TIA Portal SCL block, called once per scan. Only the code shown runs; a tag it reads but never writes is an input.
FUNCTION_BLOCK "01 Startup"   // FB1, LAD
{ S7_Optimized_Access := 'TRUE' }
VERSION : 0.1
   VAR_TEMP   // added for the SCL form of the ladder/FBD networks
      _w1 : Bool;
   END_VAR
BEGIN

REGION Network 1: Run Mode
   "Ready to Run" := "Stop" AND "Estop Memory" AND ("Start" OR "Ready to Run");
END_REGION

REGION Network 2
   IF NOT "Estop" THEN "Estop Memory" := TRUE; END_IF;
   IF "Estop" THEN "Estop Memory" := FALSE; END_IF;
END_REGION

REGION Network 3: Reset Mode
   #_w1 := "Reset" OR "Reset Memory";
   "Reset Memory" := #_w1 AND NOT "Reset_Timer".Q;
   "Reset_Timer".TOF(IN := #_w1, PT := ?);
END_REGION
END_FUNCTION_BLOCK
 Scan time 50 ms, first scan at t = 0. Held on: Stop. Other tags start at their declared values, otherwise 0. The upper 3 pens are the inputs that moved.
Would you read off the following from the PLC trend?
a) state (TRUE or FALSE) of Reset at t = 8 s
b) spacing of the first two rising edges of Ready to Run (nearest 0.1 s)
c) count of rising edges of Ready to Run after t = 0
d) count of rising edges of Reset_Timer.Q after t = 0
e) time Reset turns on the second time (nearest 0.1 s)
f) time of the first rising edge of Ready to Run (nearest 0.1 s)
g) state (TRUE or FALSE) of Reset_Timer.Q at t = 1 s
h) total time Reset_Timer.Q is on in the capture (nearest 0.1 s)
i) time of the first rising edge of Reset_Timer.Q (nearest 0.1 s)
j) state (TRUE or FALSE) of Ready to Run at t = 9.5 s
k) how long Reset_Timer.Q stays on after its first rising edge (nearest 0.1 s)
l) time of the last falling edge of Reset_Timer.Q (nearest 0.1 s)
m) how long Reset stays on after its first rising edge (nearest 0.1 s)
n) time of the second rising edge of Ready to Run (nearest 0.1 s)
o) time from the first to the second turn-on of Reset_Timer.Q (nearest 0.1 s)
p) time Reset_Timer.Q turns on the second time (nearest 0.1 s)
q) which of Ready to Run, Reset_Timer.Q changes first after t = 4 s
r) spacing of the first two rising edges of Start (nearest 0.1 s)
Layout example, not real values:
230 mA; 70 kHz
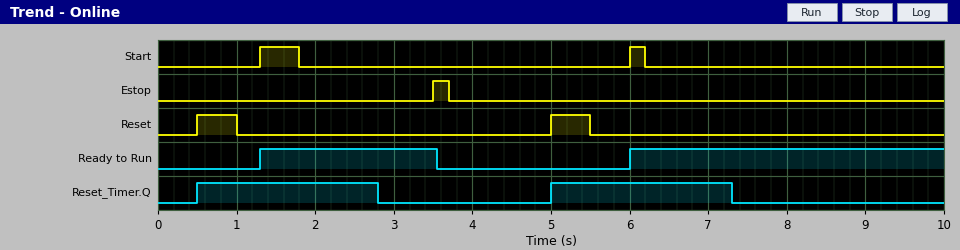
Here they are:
FALSE; 4.7 s; 2; 2; 5.0 s; 1.3 s; TRUE; 4.6 s; 0.5 s; TRUE; 2.3 s; 7.3 s; 0.5 s; 6.0 s; 4.5 s; 5.0 s; Reset_Timer.Q; 4.7 s
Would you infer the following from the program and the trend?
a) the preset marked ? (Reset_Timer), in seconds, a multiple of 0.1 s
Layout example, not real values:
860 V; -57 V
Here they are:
1.8 s
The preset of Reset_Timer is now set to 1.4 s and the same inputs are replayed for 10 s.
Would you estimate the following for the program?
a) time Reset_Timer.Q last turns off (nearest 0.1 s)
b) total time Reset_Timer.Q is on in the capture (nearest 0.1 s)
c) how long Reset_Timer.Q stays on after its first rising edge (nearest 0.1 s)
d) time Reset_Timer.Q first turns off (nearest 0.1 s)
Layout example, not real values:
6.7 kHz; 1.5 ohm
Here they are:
6.9 s; 3.8 s; 1.9 s; 2.4 s
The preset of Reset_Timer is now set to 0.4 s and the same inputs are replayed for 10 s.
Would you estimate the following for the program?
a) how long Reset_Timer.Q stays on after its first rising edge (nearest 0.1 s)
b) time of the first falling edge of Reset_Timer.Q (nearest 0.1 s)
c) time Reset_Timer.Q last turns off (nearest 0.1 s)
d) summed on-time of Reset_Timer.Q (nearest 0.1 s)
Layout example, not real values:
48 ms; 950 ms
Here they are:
0.9 s; 1.4 s; 5.9 s; 1.8 s
